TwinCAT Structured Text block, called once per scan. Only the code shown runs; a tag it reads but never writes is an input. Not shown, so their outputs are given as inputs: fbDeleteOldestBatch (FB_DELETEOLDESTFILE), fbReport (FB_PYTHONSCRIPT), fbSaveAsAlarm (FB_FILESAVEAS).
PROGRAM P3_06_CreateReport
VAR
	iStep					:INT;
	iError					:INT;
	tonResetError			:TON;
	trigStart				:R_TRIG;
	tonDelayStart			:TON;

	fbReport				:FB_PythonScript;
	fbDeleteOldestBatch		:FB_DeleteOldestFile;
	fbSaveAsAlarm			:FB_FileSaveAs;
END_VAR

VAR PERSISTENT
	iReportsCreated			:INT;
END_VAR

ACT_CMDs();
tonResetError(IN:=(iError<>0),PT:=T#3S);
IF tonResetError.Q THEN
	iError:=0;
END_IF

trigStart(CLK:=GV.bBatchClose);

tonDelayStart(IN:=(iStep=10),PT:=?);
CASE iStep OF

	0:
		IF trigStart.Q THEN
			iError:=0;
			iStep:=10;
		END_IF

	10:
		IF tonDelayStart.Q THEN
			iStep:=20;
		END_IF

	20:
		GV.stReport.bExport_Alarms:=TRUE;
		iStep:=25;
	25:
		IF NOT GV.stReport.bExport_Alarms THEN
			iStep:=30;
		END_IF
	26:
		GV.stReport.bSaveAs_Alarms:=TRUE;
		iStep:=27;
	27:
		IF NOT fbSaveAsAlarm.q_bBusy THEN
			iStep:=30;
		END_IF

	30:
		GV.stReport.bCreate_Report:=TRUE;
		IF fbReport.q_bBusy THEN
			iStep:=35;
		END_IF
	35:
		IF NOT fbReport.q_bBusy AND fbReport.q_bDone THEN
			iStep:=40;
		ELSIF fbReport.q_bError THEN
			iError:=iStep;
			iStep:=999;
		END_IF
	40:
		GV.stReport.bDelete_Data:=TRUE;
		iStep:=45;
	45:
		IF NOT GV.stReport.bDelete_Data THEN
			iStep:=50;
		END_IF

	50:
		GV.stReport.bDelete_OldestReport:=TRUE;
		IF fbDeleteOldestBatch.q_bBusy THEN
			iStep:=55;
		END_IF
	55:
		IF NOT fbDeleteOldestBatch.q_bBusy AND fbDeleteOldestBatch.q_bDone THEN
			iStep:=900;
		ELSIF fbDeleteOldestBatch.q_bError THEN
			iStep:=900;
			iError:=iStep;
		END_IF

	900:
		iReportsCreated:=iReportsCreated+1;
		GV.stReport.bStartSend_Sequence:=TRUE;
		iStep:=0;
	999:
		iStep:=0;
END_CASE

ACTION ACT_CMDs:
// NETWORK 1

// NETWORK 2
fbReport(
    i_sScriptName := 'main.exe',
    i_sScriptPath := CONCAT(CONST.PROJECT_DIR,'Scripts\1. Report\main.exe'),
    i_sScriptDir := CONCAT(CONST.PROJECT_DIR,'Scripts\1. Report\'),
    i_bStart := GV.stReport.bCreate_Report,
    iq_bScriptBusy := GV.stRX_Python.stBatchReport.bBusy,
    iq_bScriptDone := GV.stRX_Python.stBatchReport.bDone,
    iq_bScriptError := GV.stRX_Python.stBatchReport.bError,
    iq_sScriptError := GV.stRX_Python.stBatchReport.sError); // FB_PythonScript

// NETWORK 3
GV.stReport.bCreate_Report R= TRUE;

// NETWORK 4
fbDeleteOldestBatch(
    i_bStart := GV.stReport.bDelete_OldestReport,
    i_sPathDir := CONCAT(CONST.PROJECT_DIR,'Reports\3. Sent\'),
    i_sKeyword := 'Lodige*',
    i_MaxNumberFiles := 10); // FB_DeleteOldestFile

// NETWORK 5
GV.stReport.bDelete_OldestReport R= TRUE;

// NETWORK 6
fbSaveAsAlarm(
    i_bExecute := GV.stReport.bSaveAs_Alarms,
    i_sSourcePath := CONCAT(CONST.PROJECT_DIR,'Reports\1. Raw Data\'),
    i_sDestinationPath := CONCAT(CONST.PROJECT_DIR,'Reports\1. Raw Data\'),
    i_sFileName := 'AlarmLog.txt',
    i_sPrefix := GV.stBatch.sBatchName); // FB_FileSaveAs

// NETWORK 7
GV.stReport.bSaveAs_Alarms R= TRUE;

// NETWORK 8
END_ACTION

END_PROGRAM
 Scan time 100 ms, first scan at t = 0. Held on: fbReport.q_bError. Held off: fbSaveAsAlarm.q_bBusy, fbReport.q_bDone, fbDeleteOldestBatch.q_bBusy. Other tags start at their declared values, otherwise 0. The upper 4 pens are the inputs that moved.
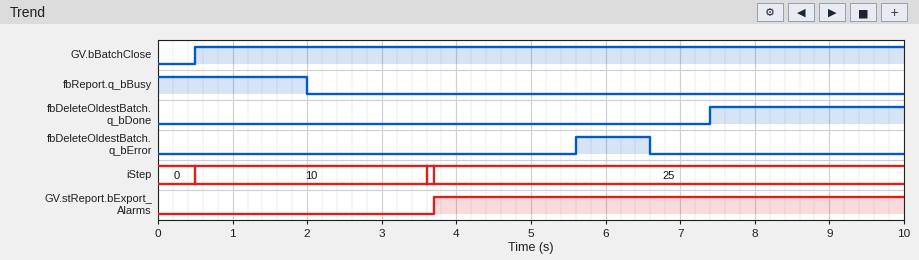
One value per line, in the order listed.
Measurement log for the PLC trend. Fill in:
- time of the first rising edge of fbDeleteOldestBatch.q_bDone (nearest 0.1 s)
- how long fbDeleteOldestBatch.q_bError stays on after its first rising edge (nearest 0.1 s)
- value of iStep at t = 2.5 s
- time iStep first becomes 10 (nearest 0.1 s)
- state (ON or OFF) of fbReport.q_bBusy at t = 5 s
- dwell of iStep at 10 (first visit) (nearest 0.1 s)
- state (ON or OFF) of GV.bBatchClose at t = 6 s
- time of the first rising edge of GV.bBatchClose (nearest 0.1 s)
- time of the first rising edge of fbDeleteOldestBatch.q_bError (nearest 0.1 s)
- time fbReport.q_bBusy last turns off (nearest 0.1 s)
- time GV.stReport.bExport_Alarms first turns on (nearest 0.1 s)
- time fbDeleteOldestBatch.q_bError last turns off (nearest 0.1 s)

7.4 s
1.0 s
10
0.5 s
OFF
3.1 s
ON
0.5 s
5.6 s
2.0 s
3.7 s
6.6 s
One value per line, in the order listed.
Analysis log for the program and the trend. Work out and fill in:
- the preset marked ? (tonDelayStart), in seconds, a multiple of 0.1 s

3.0 s
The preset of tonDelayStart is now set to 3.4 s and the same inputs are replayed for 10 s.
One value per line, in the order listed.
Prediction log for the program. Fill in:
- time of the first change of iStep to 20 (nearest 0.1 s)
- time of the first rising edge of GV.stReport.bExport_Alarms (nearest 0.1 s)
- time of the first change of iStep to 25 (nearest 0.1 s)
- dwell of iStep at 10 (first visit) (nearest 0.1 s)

4.0 s
4.1 s
4.1 s
3.5 s
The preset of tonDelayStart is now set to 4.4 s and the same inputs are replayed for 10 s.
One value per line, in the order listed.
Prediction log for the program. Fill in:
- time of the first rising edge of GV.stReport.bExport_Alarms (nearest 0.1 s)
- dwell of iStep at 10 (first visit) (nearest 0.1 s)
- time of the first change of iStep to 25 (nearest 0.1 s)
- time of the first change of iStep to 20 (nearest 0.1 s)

5.1 s
4.5 s
5.1 s
5.0 s
